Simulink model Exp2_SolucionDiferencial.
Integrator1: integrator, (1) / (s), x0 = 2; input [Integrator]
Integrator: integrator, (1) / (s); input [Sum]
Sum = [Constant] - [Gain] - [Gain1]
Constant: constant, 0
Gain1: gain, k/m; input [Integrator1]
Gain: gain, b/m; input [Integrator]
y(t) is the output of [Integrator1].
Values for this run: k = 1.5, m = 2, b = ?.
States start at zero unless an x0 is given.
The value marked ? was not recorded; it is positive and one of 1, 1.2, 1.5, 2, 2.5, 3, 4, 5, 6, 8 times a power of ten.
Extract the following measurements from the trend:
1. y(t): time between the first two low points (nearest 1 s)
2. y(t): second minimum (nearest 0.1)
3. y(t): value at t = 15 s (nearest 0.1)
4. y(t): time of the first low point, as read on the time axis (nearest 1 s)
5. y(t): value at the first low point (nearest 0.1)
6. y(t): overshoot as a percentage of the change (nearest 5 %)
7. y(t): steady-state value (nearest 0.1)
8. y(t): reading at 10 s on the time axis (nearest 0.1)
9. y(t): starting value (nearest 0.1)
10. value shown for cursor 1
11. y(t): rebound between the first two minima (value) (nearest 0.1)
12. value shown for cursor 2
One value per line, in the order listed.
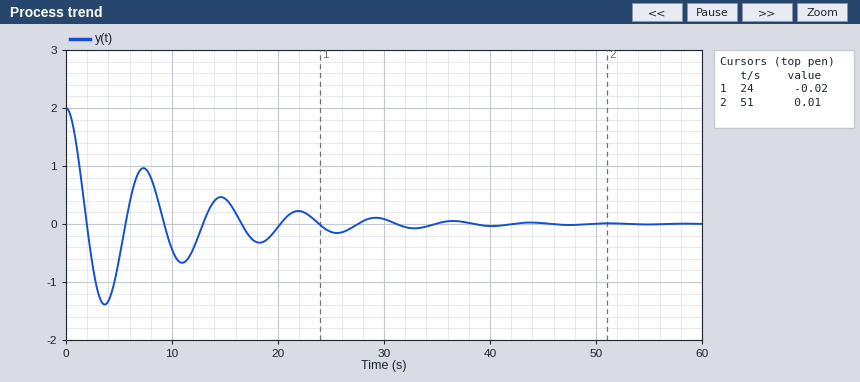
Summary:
7 s
-0.7
0.4
4 s
-1.4
70 %
0.0
-0.4
2.0
-0.02
1.0
0.01
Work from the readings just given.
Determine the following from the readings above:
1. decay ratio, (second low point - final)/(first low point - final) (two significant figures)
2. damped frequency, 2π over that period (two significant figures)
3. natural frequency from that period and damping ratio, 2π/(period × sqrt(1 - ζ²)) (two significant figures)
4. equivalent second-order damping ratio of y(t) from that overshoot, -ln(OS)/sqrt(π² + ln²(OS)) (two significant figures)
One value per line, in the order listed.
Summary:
0.50
0.90 rad/s
0.90 rad/s
0.11
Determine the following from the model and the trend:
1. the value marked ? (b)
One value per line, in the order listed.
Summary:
0.4
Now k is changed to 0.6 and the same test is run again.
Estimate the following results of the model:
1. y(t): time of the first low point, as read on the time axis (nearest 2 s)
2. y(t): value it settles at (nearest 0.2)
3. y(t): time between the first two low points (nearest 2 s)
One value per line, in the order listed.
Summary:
6 s
0.0
12 s
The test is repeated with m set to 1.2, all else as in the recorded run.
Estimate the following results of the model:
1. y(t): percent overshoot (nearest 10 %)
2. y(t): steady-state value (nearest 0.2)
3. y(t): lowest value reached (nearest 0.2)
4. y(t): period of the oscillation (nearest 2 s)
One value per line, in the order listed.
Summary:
60 %
0.0
-1.2
6 s
